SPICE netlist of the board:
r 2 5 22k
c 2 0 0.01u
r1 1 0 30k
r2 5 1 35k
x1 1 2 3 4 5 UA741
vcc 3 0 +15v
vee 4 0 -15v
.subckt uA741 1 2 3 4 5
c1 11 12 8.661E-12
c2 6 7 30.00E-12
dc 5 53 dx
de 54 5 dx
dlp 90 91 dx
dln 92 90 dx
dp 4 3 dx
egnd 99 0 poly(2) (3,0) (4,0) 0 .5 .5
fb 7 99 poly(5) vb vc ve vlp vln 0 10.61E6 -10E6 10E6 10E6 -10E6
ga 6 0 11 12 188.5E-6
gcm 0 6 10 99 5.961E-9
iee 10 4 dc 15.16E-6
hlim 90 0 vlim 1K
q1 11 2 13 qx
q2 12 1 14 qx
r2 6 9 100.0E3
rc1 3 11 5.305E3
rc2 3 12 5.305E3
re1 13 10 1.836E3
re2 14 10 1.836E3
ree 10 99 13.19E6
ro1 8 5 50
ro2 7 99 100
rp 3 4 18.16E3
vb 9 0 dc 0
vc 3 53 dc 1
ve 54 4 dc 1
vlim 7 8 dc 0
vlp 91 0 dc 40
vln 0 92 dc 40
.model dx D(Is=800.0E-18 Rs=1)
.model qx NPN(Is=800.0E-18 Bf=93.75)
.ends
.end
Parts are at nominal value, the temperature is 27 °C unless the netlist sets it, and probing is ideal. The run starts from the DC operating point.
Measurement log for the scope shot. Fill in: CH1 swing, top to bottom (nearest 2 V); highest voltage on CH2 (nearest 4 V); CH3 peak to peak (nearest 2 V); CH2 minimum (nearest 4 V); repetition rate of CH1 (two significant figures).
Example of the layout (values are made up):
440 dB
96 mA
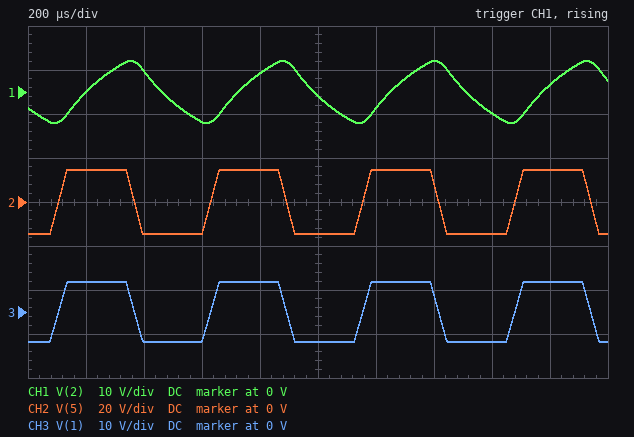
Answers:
14 V
16 V
14 V
-16 V
1.9 kHz
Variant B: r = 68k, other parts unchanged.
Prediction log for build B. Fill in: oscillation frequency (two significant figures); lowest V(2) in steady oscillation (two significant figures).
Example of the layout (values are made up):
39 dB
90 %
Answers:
690 Hz
-6.9 V
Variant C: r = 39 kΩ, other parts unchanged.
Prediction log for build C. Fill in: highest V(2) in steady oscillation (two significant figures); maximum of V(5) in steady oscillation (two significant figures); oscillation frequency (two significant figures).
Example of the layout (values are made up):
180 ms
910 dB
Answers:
6.9 V
15 V
1.2 kHz
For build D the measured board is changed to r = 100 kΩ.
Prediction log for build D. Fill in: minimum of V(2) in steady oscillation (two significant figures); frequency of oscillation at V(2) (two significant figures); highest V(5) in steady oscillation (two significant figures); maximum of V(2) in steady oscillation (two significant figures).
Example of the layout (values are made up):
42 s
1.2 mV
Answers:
-6.8 V
480 Hz
15 V
6.8 V
